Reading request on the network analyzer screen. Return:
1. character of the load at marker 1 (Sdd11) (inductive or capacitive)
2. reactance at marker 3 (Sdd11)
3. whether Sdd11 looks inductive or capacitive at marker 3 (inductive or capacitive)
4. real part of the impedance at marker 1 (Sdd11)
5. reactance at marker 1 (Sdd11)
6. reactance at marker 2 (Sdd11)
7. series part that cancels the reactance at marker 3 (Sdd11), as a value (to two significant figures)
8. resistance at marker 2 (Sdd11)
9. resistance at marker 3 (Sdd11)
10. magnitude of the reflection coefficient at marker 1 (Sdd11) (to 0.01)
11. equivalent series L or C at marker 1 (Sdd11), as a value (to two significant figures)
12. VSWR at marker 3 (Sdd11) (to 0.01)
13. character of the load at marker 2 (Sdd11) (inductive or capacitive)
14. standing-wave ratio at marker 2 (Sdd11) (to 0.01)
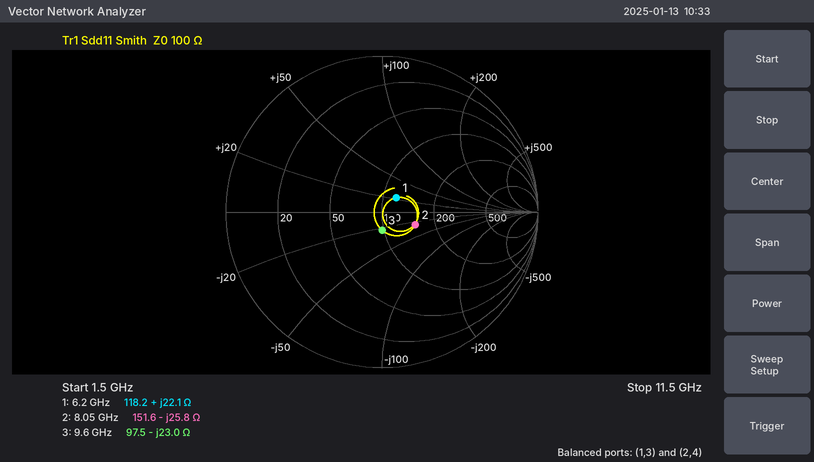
inductive
-23.0 Ω
capacitive
118.2 Ω
+22.1 Ω
-25.8 Ω
380 pH
151.6 Ω
97.5 Ω
0.13
570 pH
1.26
capacitive
1.59
